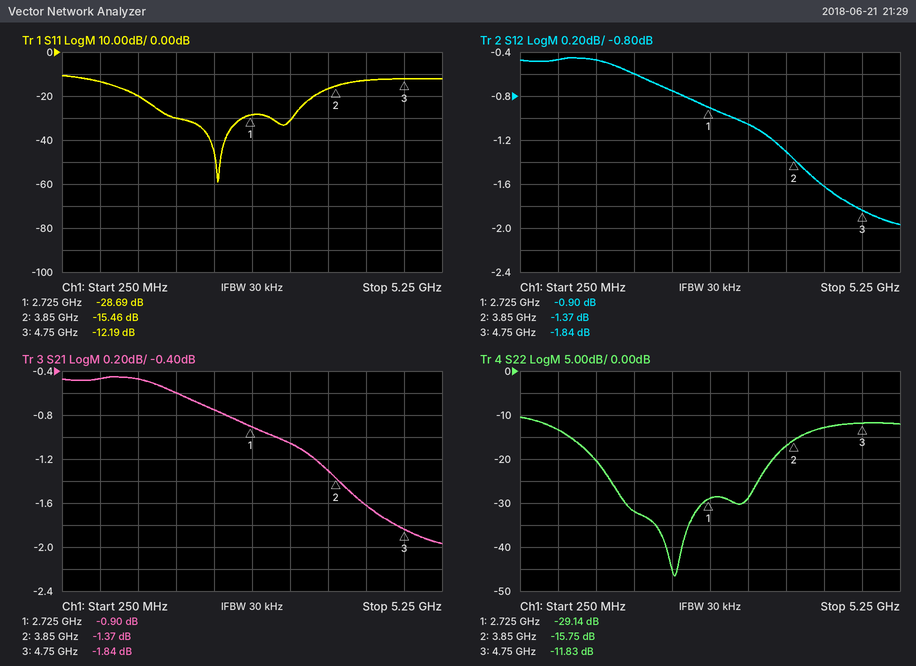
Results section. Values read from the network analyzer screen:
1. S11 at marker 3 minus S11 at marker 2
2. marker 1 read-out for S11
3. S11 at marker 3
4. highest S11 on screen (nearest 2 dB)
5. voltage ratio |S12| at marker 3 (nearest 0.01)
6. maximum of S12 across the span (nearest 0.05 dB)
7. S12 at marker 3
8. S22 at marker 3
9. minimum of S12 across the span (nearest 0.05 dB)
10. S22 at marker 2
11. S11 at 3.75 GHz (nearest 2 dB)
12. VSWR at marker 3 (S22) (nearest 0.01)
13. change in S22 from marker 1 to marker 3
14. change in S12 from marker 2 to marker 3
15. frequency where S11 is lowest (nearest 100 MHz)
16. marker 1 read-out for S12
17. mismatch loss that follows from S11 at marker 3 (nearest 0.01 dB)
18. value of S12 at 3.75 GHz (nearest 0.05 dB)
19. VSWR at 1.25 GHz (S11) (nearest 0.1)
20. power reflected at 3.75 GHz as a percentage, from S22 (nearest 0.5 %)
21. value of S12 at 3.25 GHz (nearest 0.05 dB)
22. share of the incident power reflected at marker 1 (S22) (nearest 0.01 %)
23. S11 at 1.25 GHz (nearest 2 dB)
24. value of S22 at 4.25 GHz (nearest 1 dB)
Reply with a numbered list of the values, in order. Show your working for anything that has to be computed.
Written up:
1. -12.19 − (-15.46) = 3.27 dB
2. -28.69 dB
3. -12.19 dB
4. -10 dB
5. 10^(-1.84/20) ≈ 0.81
6. -0.45 dB
7. -1.84 dB
8. -11.83 dB
9. -1.95 dB
10. -15.75 dB
11. -16 dB
12. (1 + 0.2562)/(1 − 0.2562) ≈ 1.69
13. -11.83 − (-29.14) = 17.31 dB
14. -1.84 − (-1.37) = -0.47 dB
15. 2.3 GHz
16. -0.90 dB
17. −10 log10(1 − 10^(-12.19/10)) ≈ 0.27 dB
18. -1.30 dB
19. |Γ| = 10^(-20/20) = 0.1000; VSWR = (1 + 0.1000)/(1 − 0.1000) ≈ 1.2
20. 10^(-17/10) ≈ 2.0 %
21. -1.05 dB
22. 10^(-29.14/10) ≈ 0.12 %
23. -20 dB
24. -13 dB
